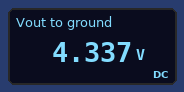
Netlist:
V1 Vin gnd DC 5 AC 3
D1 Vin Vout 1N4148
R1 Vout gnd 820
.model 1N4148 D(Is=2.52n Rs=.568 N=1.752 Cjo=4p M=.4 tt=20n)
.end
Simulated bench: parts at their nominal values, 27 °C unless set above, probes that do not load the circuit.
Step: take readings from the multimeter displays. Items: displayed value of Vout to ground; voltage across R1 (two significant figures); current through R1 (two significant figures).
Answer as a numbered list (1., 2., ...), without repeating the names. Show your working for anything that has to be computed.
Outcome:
1. 4.337 V
2. 4.337 V = 4.3 V
3. (4.337 V) / 820 Ω = 5.3 mA
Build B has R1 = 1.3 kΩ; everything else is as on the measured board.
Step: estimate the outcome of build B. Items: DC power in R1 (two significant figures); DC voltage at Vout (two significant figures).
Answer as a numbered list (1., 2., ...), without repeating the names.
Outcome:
1. 15 mW
2. 4.4 V
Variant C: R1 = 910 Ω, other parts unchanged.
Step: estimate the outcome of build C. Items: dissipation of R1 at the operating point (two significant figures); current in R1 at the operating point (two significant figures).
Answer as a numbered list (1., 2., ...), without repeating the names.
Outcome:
1. 21 mW
2. 4.8 mA
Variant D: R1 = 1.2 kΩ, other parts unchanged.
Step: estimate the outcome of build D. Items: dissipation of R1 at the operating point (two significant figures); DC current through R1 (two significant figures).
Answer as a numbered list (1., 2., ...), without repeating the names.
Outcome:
1. 16 mW
2. 3.6 mA
